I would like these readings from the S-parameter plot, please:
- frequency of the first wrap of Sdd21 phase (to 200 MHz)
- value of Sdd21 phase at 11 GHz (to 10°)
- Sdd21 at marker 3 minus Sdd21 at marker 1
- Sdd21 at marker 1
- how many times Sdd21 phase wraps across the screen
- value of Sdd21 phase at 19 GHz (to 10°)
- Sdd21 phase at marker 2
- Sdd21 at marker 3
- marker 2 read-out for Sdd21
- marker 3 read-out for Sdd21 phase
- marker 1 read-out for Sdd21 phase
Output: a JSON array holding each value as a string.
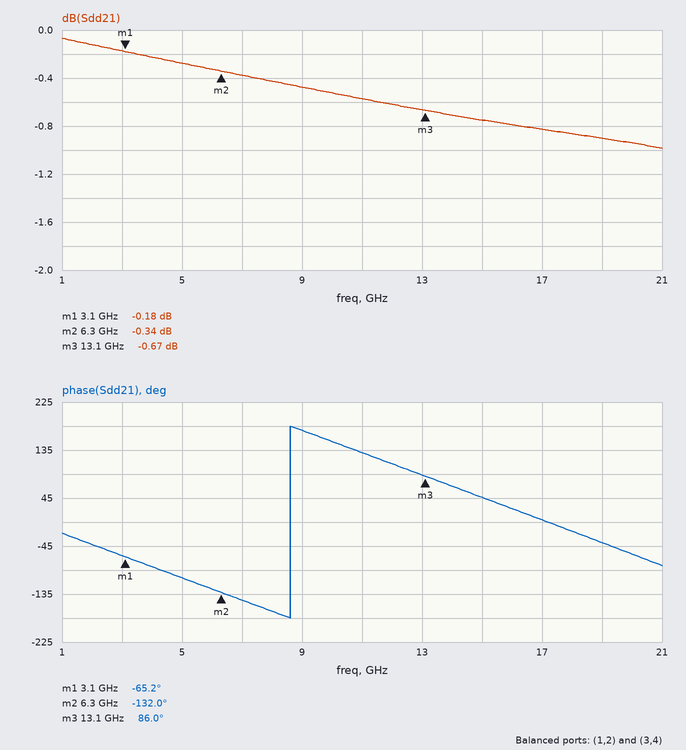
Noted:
["8.6 GHz", "130°", "-0.49 dB", "-0.18 dB", "1", "-40°", "-132.0°", "-0.67 dB", "-0.34 dB", "86.0°", "-65.2°"]
